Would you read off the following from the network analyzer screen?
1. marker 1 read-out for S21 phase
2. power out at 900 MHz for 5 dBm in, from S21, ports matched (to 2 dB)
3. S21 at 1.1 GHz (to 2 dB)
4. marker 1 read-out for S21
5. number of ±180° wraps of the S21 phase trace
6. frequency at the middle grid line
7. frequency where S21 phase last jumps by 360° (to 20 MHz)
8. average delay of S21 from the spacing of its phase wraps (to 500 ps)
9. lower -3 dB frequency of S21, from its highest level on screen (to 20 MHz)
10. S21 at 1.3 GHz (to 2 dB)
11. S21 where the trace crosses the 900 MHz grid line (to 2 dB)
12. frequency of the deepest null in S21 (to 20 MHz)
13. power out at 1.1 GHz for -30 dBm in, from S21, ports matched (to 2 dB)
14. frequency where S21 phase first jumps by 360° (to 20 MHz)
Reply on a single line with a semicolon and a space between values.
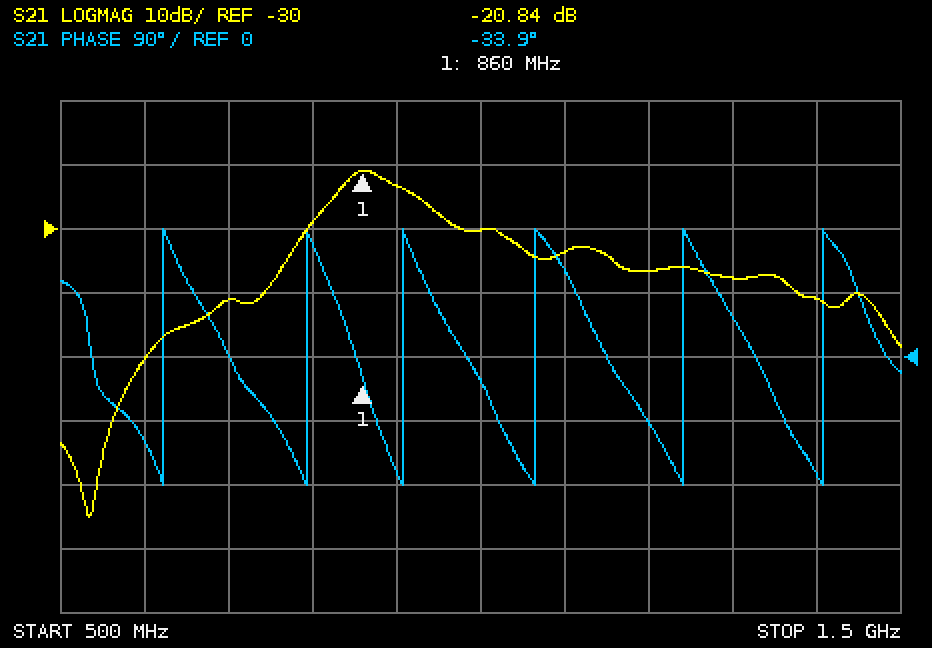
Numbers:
-33.9°; -18 dBm; -34 dB; -20.84 dB; 6; 1 GHz; 1.40 GHz; 6.5 ns; 840 MHz; -38 dB; -24 dB; 540 MHz; -64 dBm; 620 MHz
